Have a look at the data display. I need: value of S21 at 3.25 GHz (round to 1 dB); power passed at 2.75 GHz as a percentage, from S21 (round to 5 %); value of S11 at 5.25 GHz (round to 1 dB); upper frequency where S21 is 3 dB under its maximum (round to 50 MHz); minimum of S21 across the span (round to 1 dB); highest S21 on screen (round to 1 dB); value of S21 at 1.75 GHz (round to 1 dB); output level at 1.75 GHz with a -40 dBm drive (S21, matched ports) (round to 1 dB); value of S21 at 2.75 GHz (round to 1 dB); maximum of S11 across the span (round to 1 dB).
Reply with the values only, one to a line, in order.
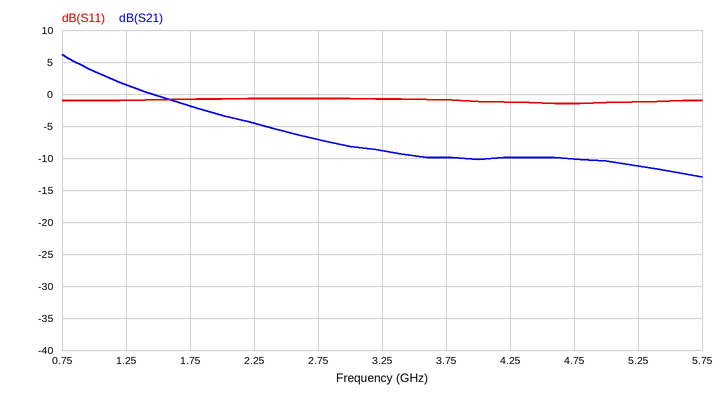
-9 dB
20 %
-1 dB
1.05 GHz
-13 dB
6 dB
-2 dB
-42 dBm
-7 dB
-1 dB
